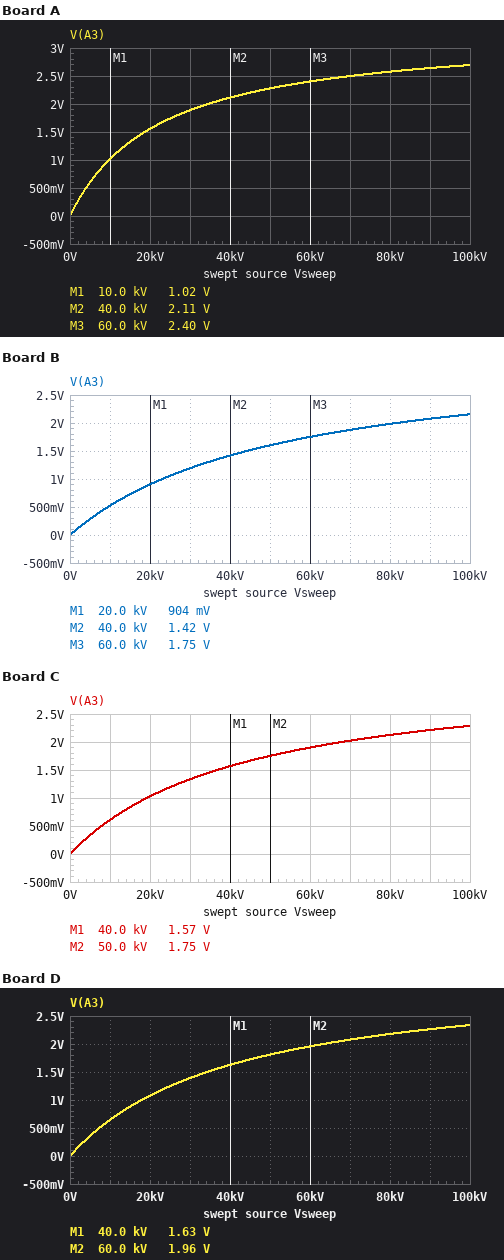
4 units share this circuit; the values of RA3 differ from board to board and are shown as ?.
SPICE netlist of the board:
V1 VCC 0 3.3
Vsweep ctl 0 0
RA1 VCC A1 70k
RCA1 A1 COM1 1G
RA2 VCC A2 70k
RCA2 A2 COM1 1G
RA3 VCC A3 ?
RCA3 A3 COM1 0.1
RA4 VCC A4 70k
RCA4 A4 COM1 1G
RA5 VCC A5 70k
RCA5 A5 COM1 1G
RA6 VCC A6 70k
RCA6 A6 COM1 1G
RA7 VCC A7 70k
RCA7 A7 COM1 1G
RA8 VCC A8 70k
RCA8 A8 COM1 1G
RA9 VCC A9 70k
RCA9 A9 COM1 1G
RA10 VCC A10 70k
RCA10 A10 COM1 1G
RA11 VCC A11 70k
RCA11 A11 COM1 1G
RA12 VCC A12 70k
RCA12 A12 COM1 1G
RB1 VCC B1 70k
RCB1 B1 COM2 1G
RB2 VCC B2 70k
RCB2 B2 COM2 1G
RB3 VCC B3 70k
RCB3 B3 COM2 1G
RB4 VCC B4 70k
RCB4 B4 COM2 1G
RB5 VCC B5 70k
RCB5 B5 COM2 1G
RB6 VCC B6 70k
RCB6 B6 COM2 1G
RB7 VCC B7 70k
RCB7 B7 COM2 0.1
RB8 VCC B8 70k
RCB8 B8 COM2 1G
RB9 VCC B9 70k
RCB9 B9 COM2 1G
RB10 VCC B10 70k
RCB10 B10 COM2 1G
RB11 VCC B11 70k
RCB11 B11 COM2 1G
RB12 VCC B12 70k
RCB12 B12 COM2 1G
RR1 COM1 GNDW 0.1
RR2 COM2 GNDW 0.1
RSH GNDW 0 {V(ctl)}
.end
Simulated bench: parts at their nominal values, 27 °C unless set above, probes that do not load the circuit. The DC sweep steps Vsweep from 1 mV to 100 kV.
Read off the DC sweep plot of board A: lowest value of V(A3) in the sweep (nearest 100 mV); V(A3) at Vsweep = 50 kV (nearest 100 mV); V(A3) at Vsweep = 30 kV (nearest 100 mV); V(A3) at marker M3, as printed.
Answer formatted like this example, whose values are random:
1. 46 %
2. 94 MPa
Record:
1. 0 V
2. 2.3 V
3. 1.9 V
4. 2.40 V
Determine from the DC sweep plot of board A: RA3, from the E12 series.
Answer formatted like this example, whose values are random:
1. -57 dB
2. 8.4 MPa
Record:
1. 33 kΩ
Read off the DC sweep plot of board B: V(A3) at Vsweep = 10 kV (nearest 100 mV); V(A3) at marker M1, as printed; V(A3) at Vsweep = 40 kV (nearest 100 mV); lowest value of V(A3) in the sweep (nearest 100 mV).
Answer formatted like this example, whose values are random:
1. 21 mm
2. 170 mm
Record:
1. 500 mV
2. 904 mV
3. 1.4 V
4. 0 V
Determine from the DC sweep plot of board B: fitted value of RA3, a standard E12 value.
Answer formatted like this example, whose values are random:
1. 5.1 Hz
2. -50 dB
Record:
1. 220 kΩ
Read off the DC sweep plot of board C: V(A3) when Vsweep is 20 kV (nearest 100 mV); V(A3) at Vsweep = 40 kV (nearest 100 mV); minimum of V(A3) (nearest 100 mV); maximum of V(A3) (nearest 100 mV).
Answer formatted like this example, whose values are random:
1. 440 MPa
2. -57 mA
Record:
1. 1.0 V
2. 1.6 V
3. 0 V
4. 2.3 V
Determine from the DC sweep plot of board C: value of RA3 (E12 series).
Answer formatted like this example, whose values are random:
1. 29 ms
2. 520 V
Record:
1. 120 kΩ
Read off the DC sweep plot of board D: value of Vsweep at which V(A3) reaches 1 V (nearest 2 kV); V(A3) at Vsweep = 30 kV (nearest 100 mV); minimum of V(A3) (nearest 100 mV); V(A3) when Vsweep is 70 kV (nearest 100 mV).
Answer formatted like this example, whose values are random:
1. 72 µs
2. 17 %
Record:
1. 18 kV
2. 1.4 V
3. 0 V
4. 2.1 V
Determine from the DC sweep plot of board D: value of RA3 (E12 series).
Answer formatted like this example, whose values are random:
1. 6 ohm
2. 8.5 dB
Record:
1. 100 kΩ
